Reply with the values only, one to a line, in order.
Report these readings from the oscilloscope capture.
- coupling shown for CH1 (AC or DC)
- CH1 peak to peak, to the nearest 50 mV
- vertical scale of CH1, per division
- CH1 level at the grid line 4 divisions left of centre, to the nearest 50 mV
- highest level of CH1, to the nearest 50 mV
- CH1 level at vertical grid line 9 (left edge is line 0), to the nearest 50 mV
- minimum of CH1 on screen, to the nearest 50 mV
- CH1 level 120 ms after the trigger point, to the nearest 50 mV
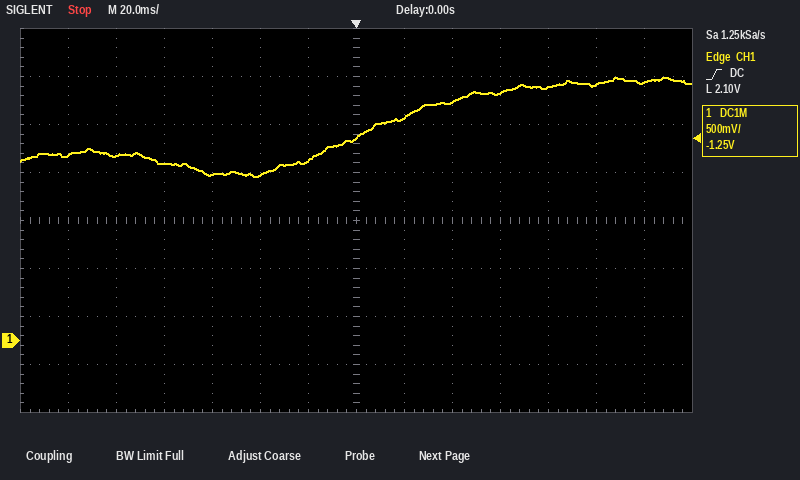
DC
1.05 V
500 mV
1.85 V
2.75 V
2.50 V
1.70 V
2.70 V
